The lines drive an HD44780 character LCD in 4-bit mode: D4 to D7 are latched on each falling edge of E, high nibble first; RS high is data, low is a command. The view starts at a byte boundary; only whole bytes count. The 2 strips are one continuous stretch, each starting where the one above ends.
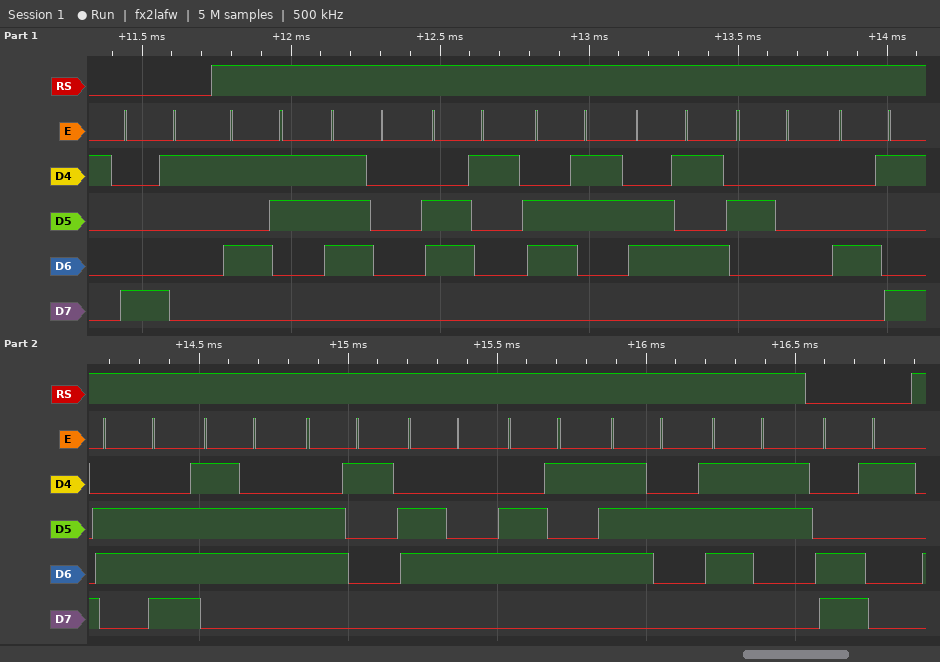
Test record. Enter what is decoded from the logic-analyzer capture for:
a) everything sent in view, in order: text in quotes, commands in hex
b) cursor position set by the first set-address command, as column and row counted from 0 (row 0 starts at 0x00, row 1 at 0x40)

0x81 "Space Invaders" 0xC1
column 1, row 0
